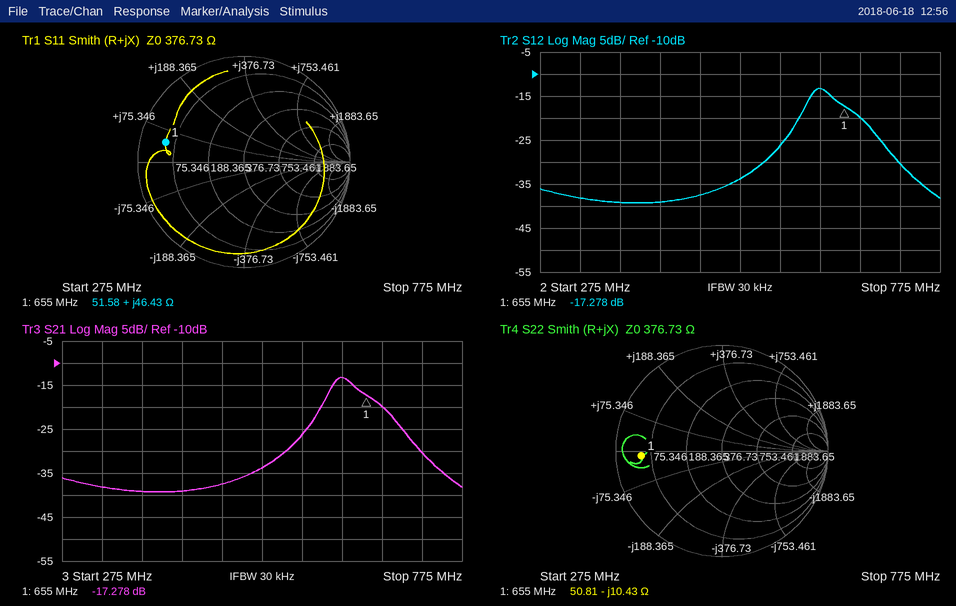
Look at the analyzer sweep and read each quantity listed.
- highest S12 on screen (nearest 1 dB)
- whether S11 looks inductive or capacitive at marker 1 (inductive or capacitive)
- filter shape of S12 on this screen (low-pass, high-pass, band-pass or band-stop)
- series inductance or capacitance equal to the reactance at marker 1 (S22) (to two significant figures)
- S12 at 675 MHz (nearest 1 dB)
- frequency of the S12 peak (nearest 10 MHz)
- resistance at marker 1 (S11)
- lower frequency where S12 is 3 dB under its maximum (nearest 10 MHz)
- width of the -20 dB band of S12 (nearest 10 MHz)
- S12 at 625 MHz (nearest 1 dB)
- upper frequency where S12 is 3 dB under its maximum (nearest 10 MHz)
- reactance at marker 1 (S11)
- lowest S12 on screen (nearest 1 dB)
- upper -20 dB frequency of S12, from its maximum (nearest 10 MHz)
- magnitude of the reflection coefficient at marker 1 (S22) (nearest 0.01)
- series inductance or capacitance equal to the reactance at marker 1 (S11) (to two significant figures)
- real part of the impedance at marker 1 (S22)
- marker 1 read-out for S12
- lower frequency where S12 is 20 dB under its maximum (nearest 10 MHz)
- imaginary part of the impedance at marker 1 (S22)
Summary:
-13 dB
inductive
band-pass
23 pF
-20 dB
620 MHz
51.58 Ω
610 MHz
210 MHz
-13 dB
650 MHz
+46.43 Ω
-39 dB
740 MHz
0.76
11 nH
50.81 Ω
-17.278 dB
530 MHz
-10.43 Ω
